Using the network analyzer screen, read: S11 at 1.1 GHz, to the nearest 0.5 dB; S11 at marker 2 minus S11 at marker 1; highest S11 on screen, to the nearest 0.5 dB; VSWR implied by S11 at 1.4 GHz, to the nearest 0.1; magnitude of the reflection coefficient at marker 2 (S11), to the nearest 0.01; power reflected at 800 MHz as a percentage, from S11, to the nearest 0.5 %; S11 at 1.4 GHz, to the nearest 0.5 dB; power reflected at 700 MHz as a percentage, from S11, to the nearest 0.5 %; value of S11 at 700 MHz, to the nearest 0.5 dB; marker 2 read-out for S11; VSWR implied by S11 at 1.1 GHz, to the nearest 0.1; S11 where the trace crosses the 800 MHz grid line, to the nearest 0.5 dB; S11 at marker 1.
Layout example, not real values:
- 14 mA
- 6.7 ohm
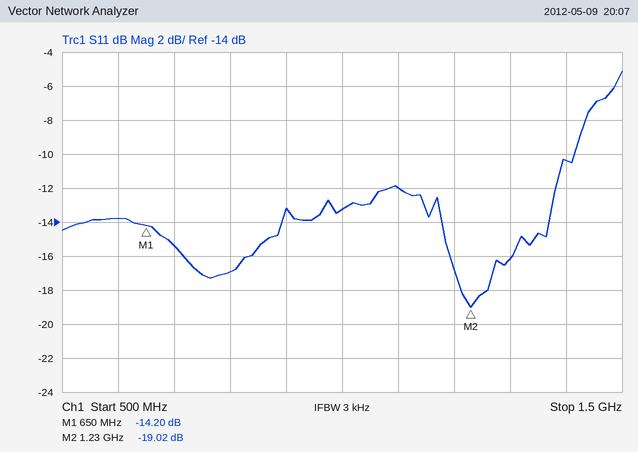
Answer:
- -12.0 dB
- -4.82 dB
- -5.0 dB
- 1.9
- 0.11
- 2.0 %
- -10.5 dB
- 3.0 %
- -15.5 dB
- -19.02 dB
- 1.7
- -17.0 dB
- -14.20 dB
